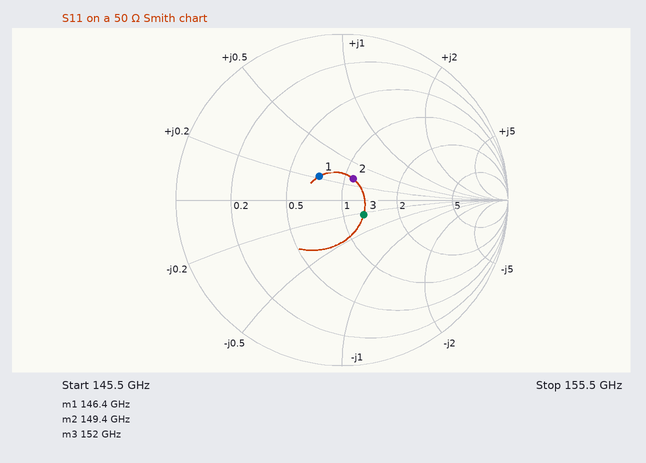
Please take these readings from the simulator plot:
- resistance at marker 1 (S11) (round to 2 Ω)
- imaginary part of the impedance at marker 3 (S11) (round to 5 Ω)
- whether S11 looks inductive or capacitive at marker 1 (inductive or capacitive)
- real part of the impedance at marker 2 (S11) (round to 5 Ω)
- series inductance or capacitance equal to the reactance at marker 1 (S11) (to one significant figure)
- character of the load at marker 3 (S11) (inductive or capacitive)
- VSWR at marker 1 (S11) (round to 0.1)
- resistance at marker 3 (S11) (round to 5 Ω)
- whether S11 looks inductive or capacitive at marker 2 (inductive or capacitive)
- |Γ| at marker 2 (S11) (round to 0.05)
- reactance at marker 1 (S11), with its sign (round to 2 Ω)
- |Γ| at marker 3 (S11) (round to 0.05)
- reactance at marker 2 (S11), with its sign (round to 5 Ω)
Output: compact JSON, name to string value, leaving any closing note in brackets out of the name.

{"resistance at marker 1 (S11)": "36 Ω", "imaginary part of the impedance at marker 3 (S11)": "-10 Ω", "whether S11 looks inductive or capacitive at marker 1": "inductive", "real part of the impedance at marker 2 (S11)": "55 Ω", "series inductance or capacitance equal to the reactance at marker 1 (S11)": "10 pH", "character of the load at marker 3 (S11)": "capacitive", "VSWR at marker 1 (S11)": "1.5", "resistance at marker 3 (S11)": "65 Ω", "whether S11 looks inductive or capacitive at marker 2": "inductive", "|Γ| at marker 2 (S11)": "0.15", "reactance at marker 1 (S11), with its sign": "+10 Ω", "|Γ| at marker 3 (S11)": "0.15", "reactance at marker 2 (S11), with its sign": "+15 Ω"}
